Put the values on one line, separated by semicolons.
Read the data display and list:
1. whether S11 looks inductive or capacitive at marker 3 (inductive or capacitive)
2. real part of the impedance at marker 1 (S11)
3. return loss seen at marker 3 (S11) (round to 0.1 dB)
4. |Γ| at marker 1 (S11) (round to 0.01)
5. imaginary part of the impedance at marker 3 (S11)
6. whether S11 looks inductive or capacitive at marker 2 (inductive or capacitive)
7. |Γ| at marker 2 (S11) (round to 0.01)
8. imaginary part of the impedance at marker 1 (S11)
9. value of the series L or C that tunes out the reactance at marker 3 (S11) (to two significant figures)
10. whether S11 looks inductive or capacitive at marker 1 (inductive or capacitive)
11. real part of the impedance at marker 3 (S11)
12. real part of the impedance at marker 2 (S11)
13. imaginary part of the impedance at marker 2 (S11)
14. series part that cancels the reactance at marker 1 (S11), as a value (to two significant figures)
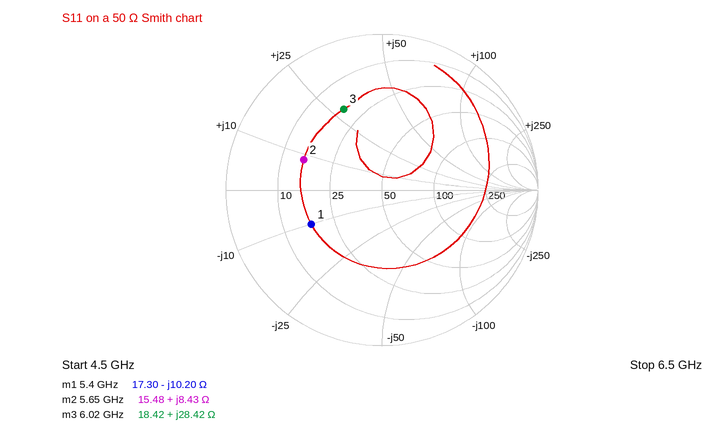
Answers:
inductive; 17.30 Ω; 4.8 dB; 0.50; +28.42 Ω; inductive; 0.54; -10.20 Ω; 930 fF; capacitive; 18.42 Ω; 15.48 Ω; +8.43 Ω; 300 pH
